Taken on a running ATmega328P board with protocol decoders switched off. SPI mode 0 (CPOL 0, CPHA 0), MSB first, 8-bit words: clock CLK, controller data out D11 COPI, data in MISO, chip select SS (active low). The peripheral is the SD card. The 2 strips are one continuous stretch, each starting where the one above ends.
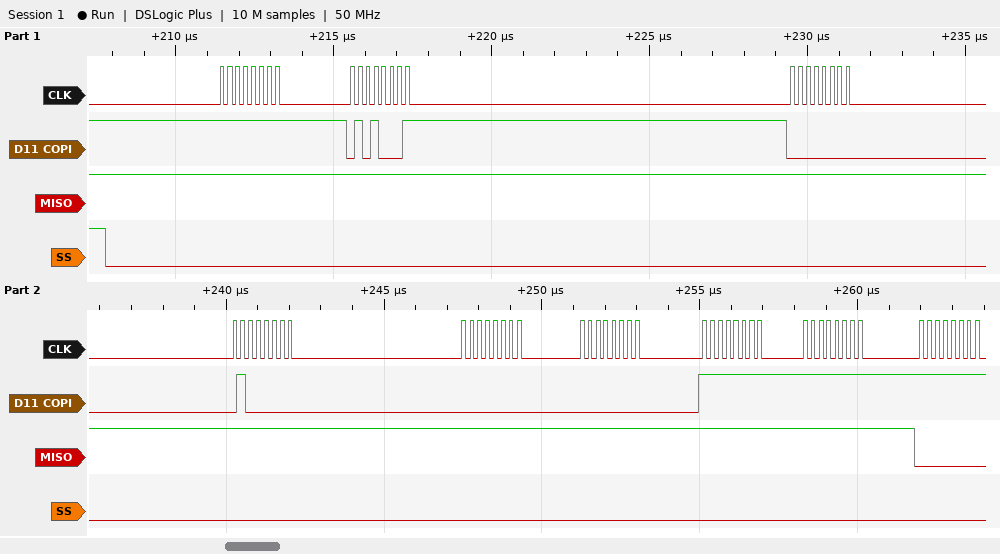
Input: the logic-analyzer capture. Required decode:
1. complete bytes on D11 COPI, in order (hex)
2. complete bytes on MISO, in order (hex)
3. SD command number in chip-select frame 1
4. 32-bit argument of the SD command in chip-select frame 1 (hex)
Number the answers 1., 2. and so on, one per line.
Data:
1. 0xFF 0x51 0x00 0x40 0x00 0x00 0xFF 0xFF 0xFF
2. 0xFF 0xFF 0xFF 0xFF 0xFF 0xFF 0xFF 0xFF 0x00
3. CMD17
4. 0x00400000
